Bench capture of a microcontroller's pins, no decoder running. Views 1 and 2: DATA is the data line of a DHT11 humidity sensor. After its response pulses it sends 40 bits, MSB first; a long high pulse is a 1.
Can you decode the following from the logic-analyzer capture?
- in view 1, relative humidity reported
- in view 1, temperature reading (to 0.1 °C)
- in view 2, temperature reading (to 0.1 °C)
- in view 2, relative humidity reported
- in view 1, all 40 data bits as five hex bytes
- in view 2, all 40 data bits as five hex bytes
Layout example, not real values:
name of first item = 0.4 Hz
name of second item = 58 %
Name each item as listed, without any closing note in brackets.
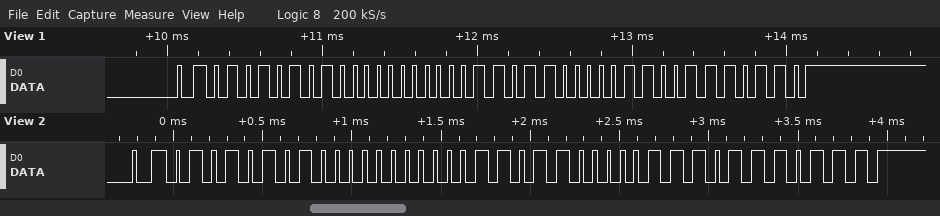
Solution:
in view 1, relative humidity reported = 85 %
in view 1, temperature reading = 27.6 °C
in view 2, temperature reading = 27.7 °C
in view 2, relative humidity reported = 85 %
in view 1, all 40 data bits as five hex bytes = 55 00 1B 06 76
in view 2, all 40 data bits as five hex bytes = 55 00 1B 07 77
